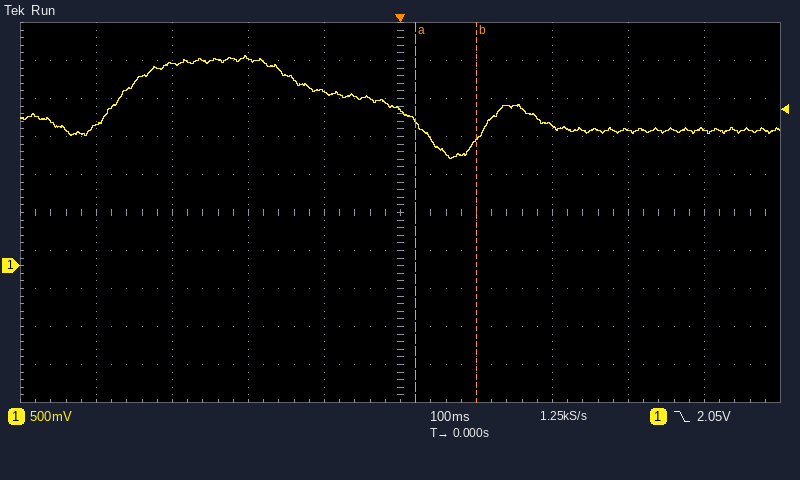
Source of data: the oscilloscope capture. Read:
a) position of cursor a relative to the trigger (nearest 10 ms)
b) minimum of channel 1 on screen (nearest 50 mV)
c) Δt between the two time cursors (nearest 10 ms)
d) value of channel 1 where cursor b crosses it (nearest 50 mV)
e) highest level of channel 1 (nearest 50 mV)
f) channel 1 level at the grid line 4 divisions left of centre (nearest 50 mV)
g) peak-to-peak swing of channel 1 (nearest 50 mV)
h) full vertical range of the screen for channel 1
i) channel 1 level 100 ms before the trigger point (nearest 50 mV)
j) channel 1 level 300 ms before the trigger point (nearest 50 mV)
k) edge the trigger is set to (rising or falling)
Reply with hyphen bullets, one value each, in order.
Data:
- +20 ms
- 1.40 V
- 80 ms
- 1.65 V
- 2.75 V
- 1.85 V
- 1.35 V
- 5 V
- 2.30 V
- 2.65 V
- falling
